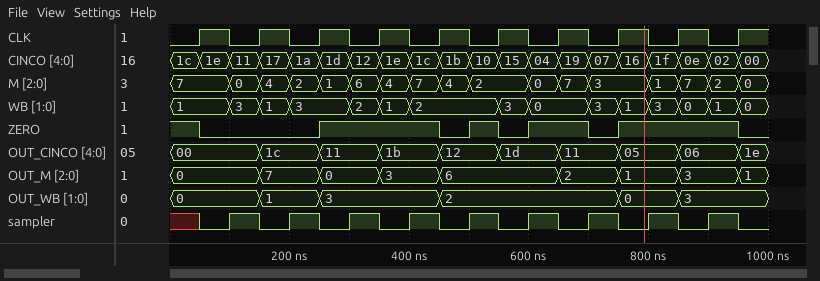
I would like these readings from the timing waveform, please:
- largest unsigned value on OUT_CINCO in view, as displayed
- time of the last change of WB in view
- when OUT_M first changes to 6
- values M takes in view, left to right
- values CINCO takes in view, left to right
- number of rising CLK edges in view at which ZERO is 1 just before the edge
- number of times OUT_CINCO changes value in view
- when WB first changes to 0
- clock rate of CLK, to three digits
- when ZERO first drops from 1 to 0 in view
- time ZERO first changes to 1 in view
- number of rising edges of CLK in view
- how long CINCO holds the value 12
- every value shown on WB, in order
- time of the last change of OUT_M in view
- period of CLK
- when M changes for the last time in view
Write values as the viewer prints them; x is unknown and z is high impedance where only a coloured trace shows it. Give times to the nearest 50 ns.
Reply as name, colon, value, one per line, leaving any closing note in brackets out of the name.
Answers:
largest unsigned value on OUT_CINCO in view, as displayed: 1e
time of the last change of WB in view: 950 ns
when OUT_M first changes to 6: 450 ns
values M takes in view, left to right: 7, 0, 4, 2, 1, 6, 4, 7, 4, 2, 0, 7, 3, 1, 7, 2, 0
values CINCO takes in view, left to right: 1c, 1e, 11, 17, 1a, 1d, 12, 1e, 1c, 1b, 10, 15, 04, 19, 07, 16, 1f, 0e, 02, 00
number of rising CLK edges in view at which ZERO is 1 just before the edge: 7
number of times OUT_CINCO changes value in view: 9
when WB first changes to 0: 600 ns
clock rate of CLK, to three digits: 10.0 MHz
when ZERO first drops from 1 to 0 in view: 50 ns
time ZERO first changes to 1 in view: 250 ns
number of rising edges of CLK in view: 10
how long CINCO holds the value 12: 50 ns
every value shown on WB, in order: 1, 3, 1, 3, 2, 1, 2, 3, 0, 3, 1, 3, 0, 1, 0
time of the last change of OUT_M in view: 950 ns
period of CLK: 100 ns
when M changes for the last time in view: 950 ns
